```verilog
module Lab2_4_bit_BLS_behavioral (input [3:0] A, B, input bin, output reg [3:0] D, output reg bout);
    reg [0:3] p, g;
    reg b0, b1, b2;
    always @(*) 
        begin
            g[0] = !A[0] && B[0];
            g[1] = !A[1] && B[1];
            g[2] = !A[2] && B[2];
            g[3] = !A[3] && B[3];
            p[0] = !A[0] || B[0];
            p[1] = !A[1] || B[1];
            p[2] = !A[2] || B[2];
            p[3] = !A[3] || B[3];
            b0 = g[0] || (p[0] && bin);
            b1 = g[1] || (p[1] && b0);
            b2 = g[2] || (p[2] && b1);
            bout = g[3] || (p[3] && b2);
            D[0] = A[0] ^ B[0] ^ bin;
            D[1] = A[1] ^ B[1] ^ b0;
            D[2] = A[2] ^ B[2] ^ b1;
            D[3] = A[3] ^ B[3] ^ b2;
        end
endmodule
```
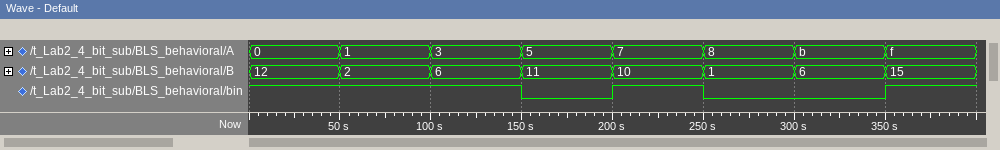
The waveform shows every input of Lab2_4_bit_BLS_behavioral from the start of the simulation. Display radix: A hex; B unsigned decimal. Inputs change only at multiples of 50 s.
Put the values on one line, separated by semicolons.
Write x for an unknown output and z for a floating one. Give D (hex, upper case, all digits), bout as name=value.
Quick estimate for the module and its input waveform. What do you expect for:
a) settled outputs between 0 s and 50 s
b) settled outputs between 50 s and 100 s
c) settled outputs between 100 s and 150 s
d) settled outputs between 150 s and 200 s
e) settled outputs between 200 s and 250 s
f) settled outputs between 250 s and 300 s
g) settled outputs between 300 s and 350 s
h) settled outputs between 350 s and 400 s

D=3, bout=1; D=E, bout=1; D=C, bout=1; D=A, bout=1; D=C, bout=1; D=7, bout=0; D=5, bout=0; D=F, bout=1
